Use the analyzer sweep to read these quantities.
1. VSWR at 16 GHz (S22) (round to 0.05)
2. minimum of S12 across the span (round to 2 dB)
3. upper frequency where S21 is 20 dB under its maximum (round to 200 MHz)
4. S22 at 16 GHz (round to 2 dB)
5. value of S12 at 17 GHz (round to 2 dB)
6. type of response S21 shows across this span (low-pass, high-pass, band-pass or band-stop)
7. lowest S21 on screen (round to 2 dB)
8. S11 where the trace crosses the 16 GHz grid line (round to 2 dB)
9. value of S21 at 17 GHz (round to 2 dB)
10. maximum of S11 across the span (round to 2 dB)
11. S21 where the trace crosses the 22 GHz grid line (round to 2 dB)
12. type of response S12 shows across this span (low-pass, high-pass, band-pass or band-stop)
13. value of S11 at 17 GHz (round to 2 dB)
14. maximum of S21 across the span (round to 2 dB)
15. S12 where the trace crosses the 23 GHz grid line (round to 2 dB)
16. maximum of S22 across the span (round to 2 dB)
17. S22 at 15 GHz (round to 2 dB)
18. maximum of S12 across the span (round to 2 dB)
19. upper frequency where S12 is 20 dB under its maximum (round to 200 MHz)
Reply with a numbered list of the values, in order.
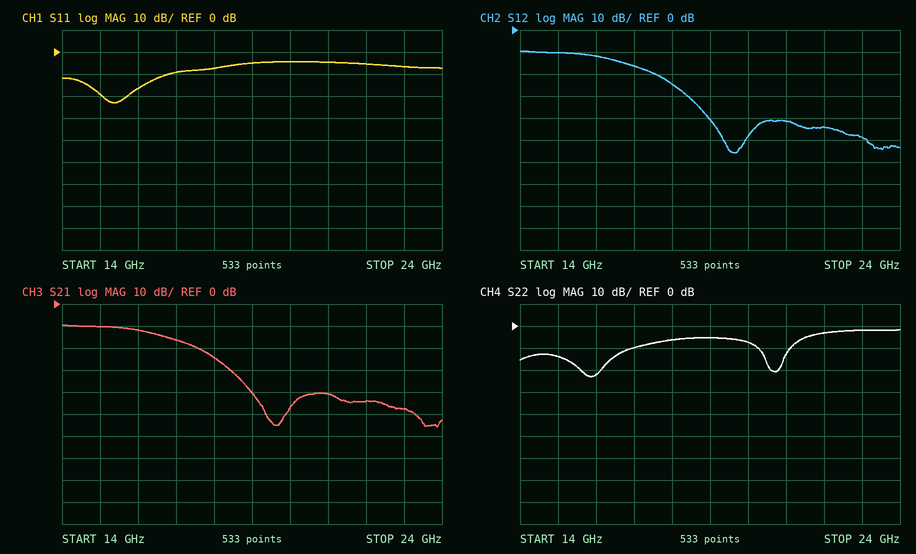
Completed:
1. 1.15
2. -56 dB
3. 18.4 GHz
4. -22 dB
5. -16 dB
6. low-pass
7. -56 dB
8. -16 dB
9. -16 dB
10. -4 dB
11. -44 dB
12. low-pass
13. -10 dB
14. -10 dB
15. -48 dB
16. -2 dB
17. -14 dB
18. -10 dB
19. 18.4 GHz
